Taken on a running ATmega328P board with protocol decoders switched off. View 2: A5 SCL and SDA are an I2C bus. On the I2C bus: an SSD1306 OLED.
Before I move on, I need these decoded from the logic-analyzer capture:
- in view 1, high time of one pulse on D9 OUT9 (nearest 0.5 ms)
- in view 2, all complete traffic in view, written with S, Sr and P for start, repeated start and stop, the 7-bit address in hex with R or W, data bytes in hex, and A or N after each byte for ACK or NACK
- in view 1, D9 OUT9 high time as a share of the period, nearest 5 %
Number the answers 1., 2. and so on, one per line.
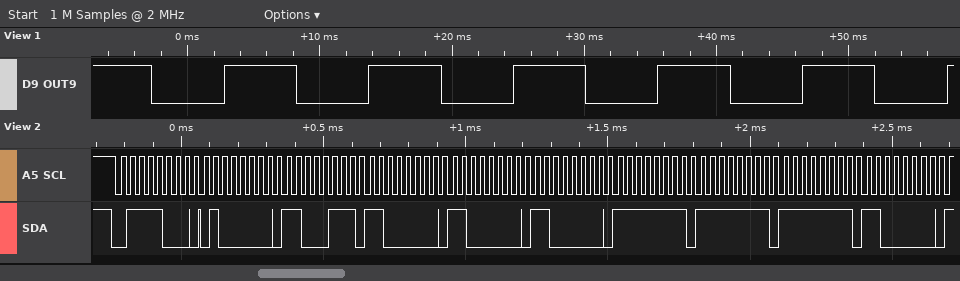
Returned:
1. 5.5 ms
2. S 3CW A 40 A C7 A C0 A C0 A C0 A FF A FF A FF A C0 A
3. 50 %
